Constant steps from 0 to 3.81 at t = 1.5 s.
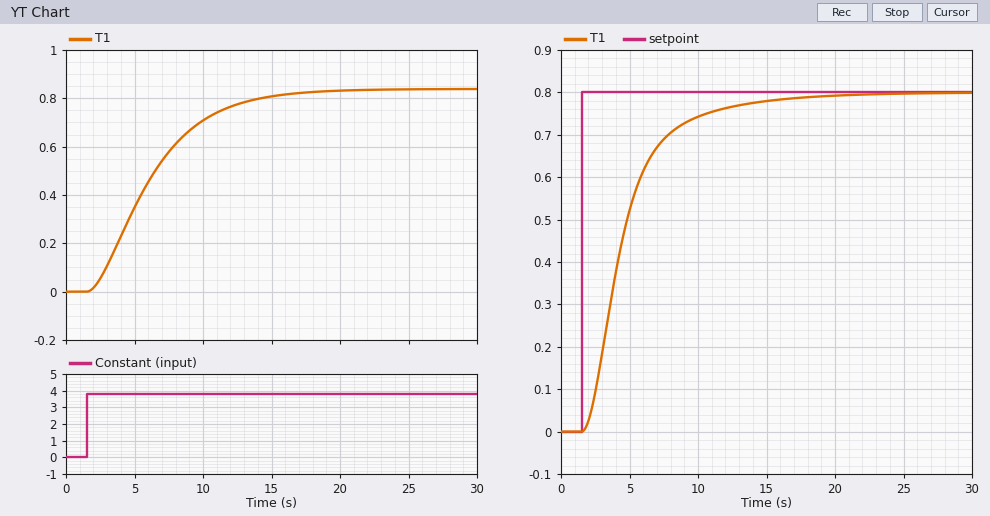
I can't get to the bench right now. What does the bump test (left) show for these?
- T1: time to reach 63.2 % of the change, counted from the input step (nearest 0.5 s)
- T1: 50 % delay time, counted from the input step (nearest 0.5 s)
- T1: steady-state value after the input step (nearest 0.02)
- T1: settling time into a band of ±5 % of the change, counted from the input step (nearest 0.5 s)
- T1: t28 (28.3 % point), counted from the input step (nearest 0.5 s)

5.5 s
4.0 s
0.84
12.5 s
2.5 s
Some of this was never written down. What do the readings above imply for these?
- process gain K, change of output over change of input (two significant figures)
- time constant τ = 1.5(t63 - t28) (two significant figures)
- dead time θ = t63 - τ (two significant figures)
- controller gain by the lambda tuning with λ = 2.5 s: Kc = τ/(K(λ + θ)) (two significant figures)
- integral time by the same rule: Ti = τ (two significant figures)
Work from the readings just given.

0.22
4.5 s
1.0 s
5.8
4.5 s
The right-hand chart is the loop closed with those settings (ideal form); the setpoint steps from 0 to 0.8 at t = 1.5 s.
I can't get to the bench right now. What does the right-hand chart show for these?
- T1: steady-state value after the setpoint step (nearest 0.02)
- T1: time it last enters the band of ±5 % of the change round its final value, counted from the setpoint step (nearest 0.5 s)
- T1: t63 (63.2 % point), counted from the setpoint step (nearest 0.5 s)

0.80
10.0 s
3.5 s
